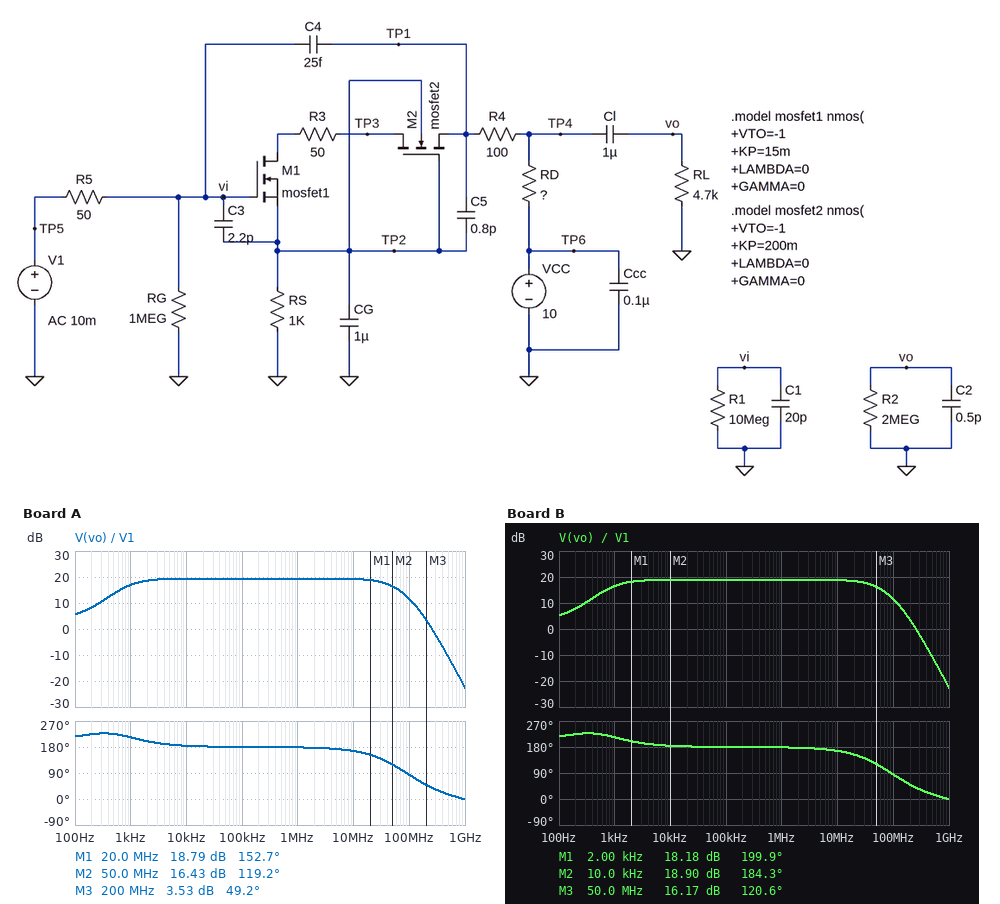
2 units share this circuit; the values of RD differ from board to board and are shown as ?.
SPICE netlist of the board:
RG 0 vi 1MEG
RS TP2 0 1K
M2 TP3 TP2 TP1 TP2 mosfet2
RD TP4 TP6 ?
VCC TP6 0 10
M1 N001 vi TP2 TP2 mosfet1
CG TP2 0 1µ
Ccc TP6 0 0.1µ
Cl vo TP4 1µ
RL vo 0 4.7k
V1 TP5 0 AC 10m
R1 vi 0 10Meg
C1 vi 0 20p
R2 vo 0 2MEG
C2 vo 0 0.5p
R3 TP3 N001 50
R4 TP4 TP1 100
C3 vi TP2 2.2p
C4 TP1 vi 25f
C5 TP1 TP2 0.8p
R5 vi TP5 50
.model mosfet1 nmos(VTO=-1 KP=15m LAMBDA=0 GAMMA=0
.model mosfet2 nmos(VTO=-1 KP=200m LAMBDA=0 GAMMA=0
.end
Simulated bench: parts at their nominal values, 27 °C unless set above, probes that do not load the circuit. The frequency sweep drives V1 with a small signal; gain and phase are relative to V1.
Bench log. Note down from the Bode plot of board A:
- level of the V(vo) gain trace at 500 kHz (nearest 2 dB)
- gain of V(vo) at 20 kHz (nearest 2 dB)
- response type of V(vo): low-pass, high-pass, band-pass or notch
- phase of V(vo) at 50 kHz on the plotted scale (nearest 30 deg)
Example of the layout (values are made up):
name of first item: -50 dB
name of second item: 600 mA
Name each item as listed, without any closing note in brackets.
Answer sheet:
level of the V(vo) gain trace at 500 kHz: 20 dB
gain of V(vo) at 20 kHz: 20 dB
response type of V(vo): low-pass, high-pass, band-pass or notch: band-pass
phase of V(vo) at 50 kHz on the plotted scale: 180 deg
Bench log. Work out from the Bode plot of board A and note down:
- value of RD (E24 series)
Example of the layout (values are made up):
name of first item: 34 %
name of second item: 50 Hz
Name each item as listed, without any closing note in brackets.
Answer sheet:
value of RD: 3.6 kΩ
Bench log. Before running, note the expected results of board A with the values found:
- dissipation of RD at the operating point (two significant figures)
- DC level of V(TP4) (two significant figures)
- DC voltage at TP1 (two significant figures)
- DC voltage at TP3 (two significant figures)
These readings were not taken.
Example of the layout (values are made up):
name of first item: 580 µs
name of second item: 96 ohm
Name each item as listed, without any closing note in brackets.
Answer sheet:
dissipation of RD at the operating point: 1.7 mW
DC level of V(TP4): 7.5 V
DC voltage at TP1: 7.4 V
DC voltage at TP3: 1.6 V
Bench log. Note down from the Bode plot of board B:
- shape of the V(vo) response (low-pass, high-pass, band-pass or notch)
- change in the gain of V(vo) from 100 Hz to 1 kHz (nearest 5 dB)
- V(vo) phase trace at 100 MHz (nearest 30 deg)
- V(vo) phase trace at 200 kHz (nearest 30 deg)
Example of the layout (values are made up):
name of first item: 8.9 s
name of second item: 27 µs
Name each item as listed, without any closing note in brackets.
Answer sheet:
shape of the V(vo) response: band-pass
change in the gain of V(vo) from 100 Hz to 1 kHz: 10 dB
V(vo) phase trace at 100 MHz: 90 deg
V(vo) phase trace at 200 kHz: 180 deg
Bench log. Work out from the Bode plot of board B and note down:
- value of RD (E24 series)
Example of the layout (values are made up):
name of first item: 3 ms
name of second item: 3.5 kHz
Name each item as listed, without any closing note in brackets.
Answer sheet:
value of RD: 3.3 kΩ
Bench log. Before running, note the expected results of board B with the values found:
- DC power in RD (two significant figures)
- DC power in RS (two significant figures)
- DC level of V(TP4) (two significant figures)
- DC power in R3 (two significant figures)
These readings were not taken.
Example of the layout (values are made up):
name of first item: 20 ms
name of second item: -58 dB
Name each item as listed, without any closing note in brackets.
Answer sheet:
DC power in RD: 1.6 mW
DC power in RS: 480 µW
DC level of V(TP4): 7.7 V
DC power in R3: 24 µW
